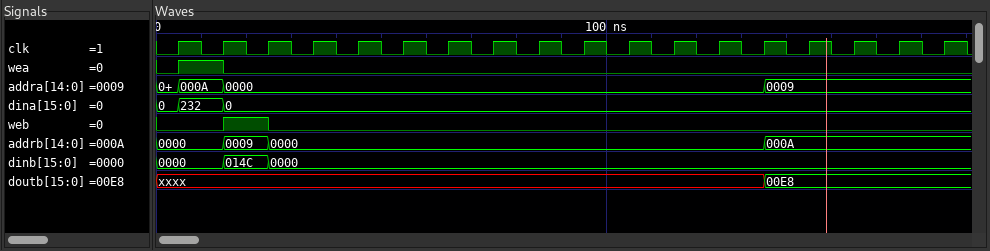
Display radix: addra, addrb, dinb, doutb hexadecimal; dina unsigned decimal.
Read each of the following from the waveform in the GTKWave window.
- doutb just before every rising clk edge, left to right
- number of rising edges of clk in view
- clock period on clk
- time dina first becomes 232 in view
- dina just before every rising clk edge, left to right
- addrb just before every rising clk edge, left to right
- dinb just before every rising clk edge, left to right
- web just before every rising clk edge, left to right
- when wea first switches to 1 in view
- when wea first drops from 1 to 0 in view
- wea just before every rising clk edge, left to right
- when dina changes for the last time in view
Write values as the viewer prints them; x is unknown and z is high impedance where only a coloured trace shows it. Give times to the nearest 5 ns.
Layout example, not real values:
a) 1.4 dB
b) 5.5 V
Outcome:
a) xxxx, xxxx, xxxx, xxxx, xxxx, xxxx, xxxx, xxxx, xxxx, xxxx, xxxx, xxxx, xxxx, xxxx, 00E8, 00E8, 00E8, 00E8
b) 18
c) 10 ns
d) 5 ns
e) 0, 232, 0, 0, 0, 0, 0, 0, 0, 0, 0, 0, 0, 0, 0, 0, 0, 0
f) 0000, 0000, 0009, 0000, 0000, 0000, 0000, 0000, 0000, 0000, 0000, 0000, 0000, 0000, 000A, 000A, 000A, 000A
g) 0000, 0000, 014C, 0000, 0000, 0000, 0000, 0000, 0000, 0000, 0000, 0000, 0000, 0000, 0000, 0000, 0000, 0000
h) 0 0 1 0 0 0 0 0 0 0 0 0 0 0 0 0 0 0
i) 5 ns
j) 15 ns
k) 0 1 0 0 0 0 0 0 0 0 0 0 0 0 0 0 0 0
l) 15 ns
